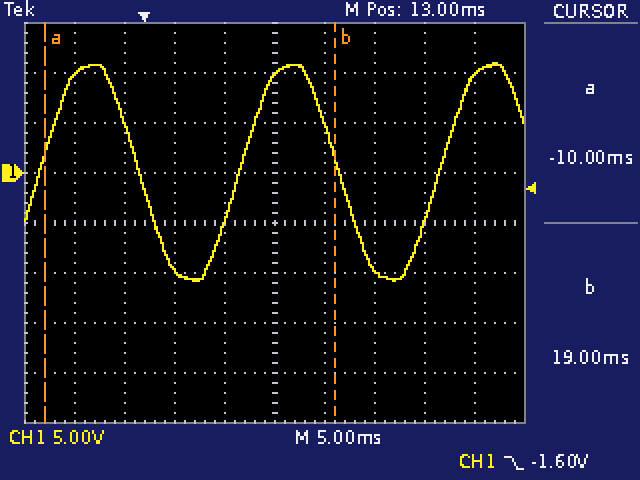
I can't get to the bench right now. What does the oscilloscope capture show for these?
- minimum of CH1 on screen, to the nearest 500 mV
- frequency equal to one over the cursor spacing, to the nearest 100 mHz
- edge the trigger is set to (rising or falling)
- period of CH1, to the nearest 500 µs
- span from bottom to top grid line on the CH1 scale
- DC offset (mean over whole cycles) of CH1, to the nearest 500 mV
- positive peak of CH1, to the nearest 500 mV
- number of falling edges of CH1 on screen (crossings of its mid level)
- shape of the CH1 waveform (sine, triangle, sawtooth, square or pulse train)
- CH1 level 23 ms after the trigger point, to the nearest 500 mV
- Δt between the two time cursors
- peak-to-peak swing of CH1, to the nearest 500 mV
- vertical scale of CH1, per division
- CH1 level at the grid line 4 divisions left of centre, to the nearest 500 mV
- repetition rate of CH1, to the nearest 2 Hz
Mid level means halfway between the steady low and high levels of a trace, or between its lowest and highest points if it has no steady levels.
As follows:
-11.0 V
34.5 Hz
falling
20.0 ms
40 V
0.0 V
11.0 V
2
sine
-9.5 V
29.0 ms
22.0 V
5 V
10.0 V
50 Hz
